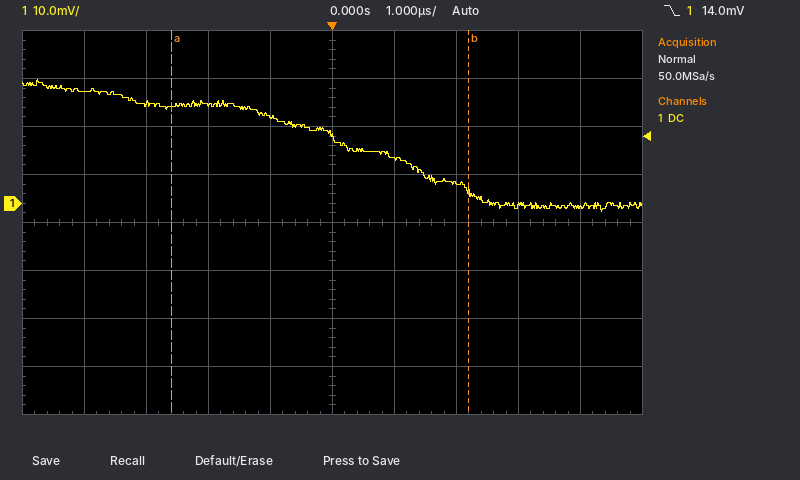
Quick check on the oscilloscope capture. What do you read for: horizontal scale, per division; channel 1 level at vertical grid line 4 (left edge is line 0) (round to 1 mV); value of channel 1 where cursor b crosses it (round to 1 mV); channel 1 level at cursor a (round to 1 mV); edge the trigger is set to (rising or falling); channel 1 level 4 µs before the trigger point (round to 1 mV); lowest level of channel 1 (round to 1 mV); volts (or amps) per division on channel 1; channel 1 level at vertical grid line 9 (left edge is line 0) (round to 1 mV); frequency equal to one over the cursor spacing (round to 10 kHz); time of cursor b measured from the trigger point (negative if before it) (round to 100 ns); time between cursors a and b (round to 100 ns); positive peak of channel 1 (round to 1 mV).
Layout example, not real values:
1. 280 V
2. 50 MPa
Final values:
1. 1 µs
2. 18 mV
3. 2 mV
4. 20 mV
5. falling
6. 23 mV
7. -2 mV
8. 10 mV
9. -1 mV
10. 210 kHz
11. +2.2 µs
12. 4.8 µs
13. 26 mV
